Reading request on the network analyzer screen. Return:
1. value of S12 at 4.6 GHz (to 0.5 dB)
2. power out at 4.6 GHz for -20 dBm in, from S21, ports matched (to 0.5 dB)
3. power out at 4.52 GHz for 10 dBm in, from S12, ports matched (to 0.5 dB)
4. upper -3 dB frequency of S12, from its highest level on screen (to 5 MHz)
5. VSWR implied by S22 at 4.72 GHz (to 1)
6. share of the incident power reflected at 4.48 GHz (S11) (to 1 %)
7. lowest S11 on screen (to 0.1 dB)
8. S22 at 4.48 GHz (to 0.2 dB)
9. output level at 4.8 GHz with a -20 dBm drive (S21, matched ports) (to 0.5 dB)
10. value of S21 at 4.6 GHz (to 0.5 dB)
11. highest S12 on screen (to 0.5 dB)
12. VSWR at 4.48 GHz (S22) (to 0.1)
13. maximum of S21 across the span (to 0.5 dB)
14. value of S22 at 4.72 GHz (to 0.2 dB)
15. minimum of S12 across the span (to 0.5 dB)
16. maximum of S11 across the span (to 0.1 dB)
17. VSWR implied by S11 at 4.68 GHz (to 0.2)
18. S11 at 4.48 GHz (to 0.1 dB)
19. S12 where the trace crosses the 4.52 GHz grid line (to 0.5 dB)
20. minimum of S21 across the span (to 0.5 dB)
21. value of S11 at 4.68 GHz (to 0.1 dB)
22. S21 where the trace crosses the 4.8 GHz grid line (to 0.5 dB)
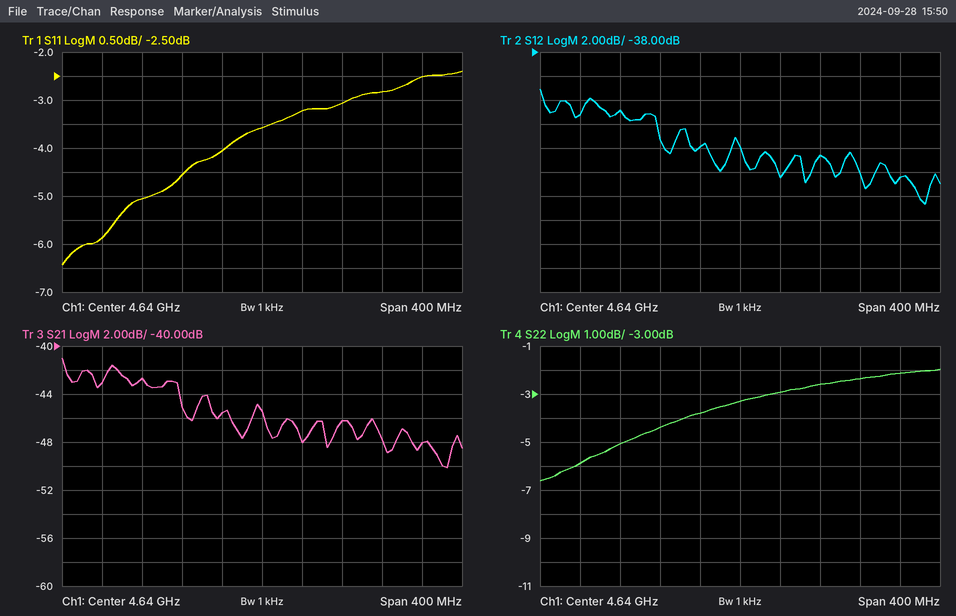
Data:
-46.0 dB
-65.5 dBm
-33.0 dBm
4.555 GHz
7
26 %
-6.4 dB
-5.8 dB
-68.0 dBm
-45.5 dB
-41.0 dB
3.1
-41.0 dB
-2.6 dB
-50.5 dB
-2.4 dB
5.4
-5.9 dB
-43.0 dB
-50.0 dB
-3.2 dB
-48.0 dB
